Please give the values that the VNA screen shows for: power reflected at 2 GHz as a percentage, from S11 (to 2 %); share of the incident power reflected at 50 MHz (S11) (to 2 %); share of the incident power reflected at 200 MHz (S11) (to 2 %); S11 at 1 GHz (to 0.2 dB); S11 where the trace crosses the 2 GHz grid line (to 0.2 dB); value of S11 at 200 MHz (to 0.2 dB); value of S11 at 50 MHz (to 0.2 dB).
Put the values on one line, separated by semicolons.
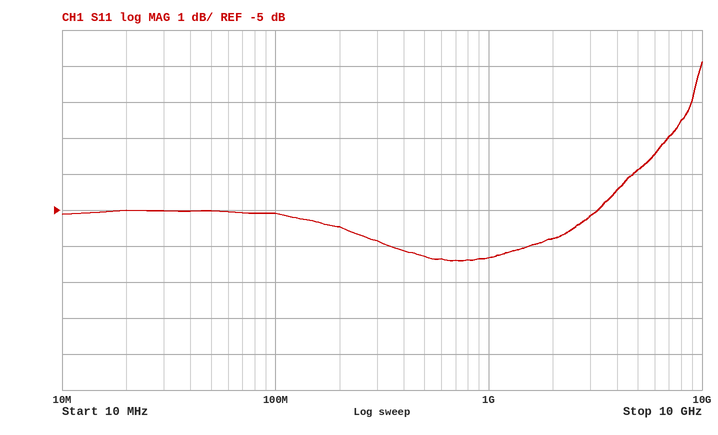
26 %; 32 %; 28 %; -6.4 dB; -5.8 dB; -5.4 dB; -5.0 dB
